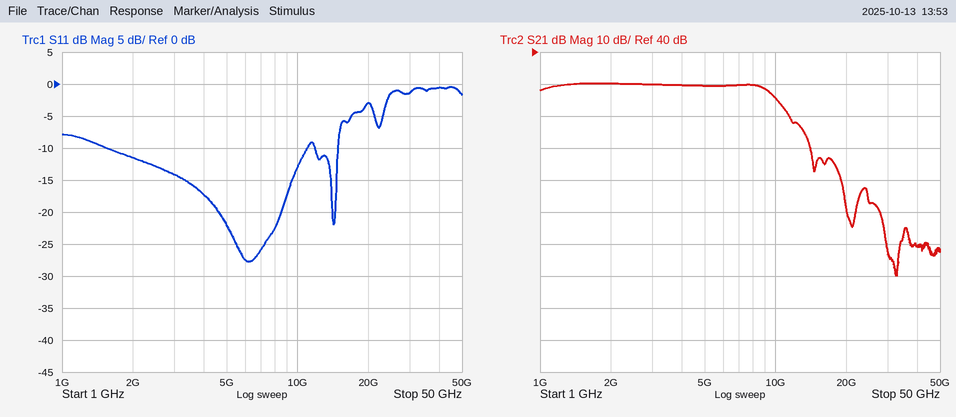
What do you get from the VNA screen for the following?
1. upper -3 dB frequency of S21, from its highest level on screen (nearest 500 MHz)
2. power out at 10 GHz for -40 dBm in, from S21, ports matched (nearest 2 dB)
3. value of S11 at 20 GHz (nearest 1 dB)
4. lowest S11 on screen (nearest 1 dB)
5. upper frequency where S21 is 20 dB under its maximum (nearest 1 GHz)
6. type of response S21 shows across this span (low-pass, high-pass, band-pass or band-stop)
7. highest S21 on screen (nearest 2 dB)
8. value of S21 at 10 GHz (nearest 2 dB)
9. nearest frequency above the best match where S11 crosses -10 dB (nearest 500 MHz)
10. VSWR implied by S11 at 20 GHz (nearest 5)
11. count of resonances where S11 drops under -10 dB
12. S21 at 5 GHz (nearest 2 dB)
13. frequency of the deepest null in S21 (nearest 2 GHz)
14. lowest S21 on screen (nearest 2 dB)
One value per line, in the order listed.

9.5 GHz
-14 dBm
-3 dB
-28 dB
14 GHz
low-pass
30 dB
26 dB
11.0 GHz
5
2
30 dB
32 GHz
-30 dB
